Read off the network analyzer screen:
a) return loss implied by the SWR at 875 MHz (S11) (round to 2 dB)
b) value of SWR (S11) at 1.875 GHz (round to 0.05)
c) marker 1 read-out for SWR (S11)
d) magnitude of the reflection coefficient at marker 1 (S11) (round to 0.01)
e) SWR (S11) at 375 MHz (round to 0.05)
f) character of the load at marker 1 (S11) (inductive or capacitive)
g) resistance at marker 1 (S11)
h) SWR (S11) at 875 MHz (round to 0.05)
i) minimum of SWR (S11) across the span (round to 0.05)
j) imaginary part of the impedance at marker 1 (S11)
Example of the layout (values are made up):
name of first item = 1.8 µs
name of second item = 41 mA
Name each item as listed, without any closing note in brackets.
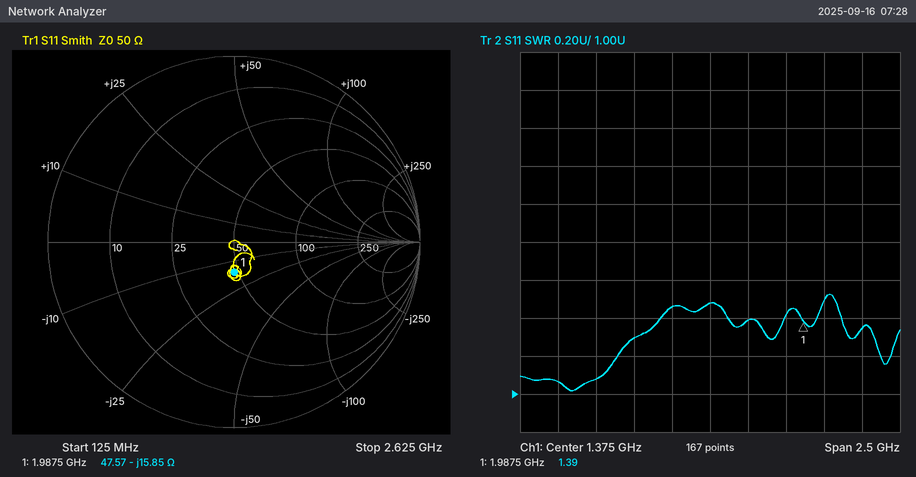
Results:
return loss implied by the SWR at 875 MHz (S11) = 18 dB
value of SWR (S11) at 1.875 GHz = 1.40
marker 1 read-out for SWR = 1.39
magnitude of the reflection coefficient at marker 1 (S11) = 0.16
SWR (S11) at 375 MHz = 1.05
character of the load at marker 1 (S11) = capacitive
resistance at marker 1 = 47.57 Ω
SWR (S11) at 875 MHz = 1.30
minimum of SWR (S11) across the span = 1.00
imaginary part of the impedance at marker 1 = -15.85 Ω
